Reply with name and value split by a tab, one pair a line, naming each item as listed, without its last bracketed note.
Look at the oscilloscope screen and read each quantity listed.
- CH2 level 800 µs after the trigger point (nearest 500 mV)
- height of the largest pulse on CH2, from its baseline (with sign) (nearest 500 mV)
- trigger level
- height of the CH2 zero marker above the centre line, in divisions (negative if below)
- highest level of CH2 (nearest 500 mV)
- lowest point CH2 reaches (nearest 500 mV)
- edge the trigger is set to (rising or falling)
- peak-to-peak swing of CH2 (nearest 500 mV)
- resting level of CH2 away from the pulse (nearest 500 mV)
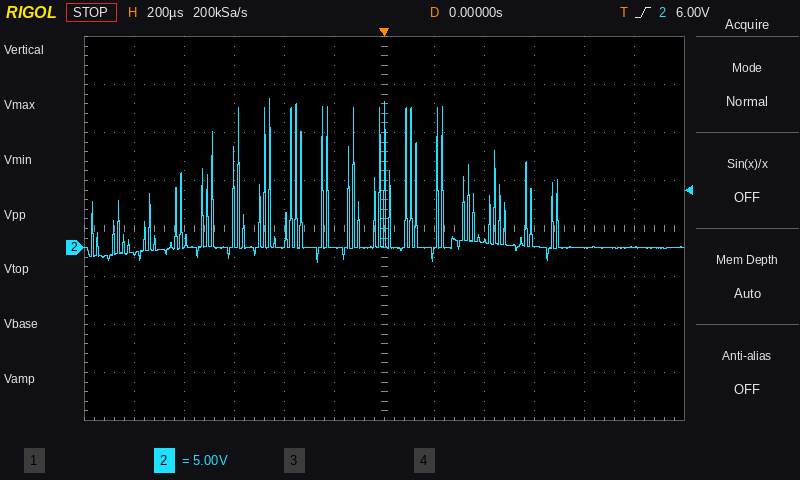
CH2 level 800 µs after the trigger point	0.0 V
height of the largest pulse on CH2, from its baseline (with sign)	+15.5 V
trigger level	6.00 V
height of the CH2 zero marker above the centre line, in divisions	-0.4 div
highest level of CH2	15.5 V
lowest point CH2 reaches	-1.5 V
edge the trigger is set to	rising
peak-to-peak swing of CH2	17.0 V
resting level of CH2 away from the pulse	0.0 V
